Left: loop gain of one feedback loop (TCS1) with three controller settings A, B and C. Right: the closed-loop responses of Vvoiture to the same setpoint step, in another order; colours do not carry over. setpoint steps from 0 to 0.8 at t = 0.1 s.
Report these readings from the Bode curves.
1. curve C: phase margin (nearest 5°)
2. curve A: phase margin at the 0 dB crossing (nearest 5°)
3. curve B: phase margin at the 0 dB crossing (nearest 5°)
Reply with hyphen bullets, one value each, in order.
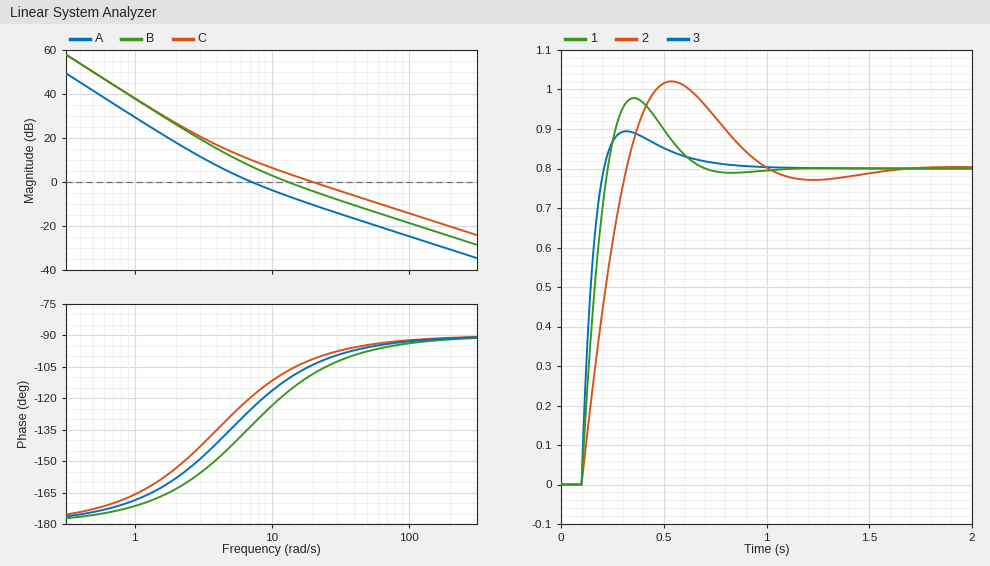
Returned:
- 80°
- 55°
- 65°
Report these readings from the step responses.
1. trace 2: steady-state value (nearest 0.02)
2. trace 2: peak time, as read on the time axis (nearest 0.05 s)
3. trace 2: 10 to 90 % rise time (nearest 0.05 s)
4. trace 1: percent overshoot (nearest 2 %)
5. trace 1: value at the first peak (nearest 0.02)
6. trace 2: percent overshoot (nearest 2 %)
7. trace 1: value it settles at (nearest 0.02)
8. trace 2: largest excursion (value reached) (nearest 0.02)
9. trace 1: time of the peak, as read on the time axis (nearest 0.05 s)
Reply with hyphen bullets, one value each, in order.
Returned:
- 0.80
- 0.55 s
- 0.15 s
- 22 %
- 0.98
- 28 %
- 0.80
- 1.02
- 0.35 s
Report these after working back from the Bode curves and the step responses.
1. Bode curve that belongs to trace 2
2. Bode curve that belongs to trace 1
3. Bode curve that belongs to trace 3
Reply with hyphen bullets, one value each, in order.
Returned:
- A
- B
- C
